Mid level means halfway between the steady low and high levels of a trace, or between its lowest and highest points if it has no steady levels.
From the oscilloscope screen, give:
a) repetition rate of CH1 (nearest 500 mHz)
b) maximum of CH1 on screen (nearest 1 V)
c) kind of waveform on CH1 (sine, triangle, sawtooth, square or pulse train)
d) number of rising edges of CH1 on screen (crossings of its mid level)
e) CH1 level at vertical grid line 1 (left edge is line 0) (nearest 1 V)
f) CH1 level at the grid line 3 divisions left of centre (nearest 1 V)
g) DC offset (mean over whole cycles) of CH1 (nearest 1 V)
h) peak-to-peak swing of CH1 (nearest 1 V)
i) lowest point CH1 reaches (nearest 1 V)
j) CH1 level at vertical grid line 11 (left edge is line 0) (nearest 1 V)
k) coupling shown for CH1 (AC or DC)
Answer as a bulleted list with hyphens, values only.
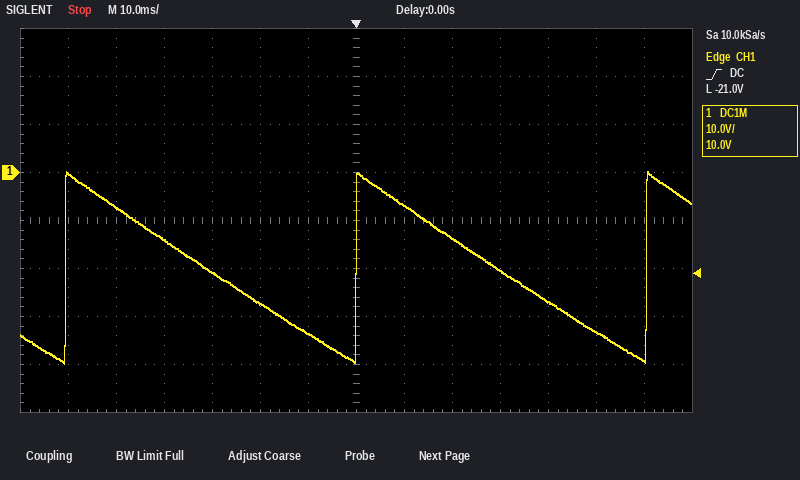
- 16.5 Hz
- 0 V
- sawtooth
- 3
- 0 V
- -21 V
- -20 V
- 40 V
- -40 V
- -27 V
- DC
